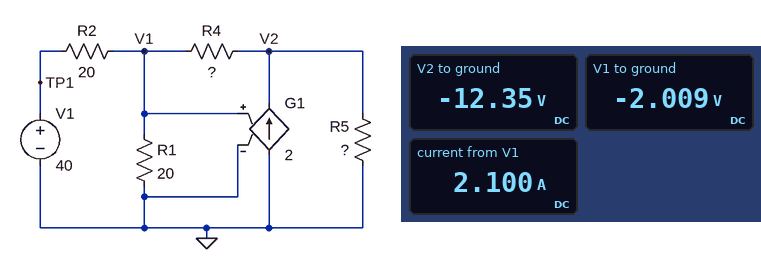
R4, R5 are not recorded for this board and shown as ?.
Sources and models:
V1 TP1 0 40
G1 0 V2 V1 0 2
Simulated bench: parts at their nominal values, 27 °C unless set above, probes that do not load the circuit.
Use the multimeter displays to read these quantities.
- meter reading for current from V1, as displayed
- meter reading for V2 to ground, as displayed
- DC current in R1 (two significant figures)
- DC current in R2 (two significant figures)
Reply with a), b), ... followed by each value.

a) 2.100 A
b) -12.35 V
c) 100 mA
d) 2.1 A
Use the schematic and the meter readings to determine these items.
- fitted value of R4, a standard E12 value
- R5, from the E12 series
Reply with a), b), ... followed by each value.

a) 4.7 Ω
b) 6.8 Ω
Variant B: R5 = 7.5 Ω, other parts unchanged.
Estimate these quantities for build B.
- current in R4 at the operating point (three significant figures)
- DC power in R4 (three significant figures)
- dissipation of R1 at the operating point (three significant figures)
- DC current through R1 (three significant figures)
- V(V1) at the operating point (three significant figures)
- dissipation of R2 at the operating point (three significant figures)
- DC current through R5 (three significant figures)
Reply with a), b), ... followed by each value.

a) 2.19 A
b) 22.6 W
c) 182 mW
d) 95.5 mA
e) -1.91 V
f) 87.8 W
g) 1.63 A
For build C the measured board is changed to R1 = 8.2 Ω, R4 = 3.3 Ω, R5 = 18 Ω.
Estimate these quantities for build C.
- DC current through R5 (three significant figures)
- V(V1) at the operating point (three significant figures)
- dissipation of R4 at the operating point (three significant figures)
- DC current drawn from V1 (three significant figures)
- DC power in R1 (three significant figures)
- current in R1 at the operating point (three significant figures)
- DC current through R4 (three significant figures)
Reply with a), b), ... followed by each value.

a) 485 mA
b) -1.36 V
c) 16.5 W
d) 2.07 A
e) 225 mW
f) 166 mA
g) 2.23 A
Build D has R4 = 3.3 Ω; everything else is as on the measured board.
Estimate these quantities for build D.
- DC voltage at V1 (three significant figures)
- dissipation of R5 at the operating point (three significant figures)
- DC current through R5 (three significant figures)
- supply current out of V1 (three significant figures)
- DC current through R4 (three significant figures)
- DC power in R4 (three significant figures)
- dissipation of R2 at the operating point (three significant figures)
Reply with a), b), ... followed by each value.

a) -1.74 V
b) 11.7 W
c) 1.31 A
d) 2.09 A
e) 2.17 A
f) 15.6 W
g) 87.1 W
